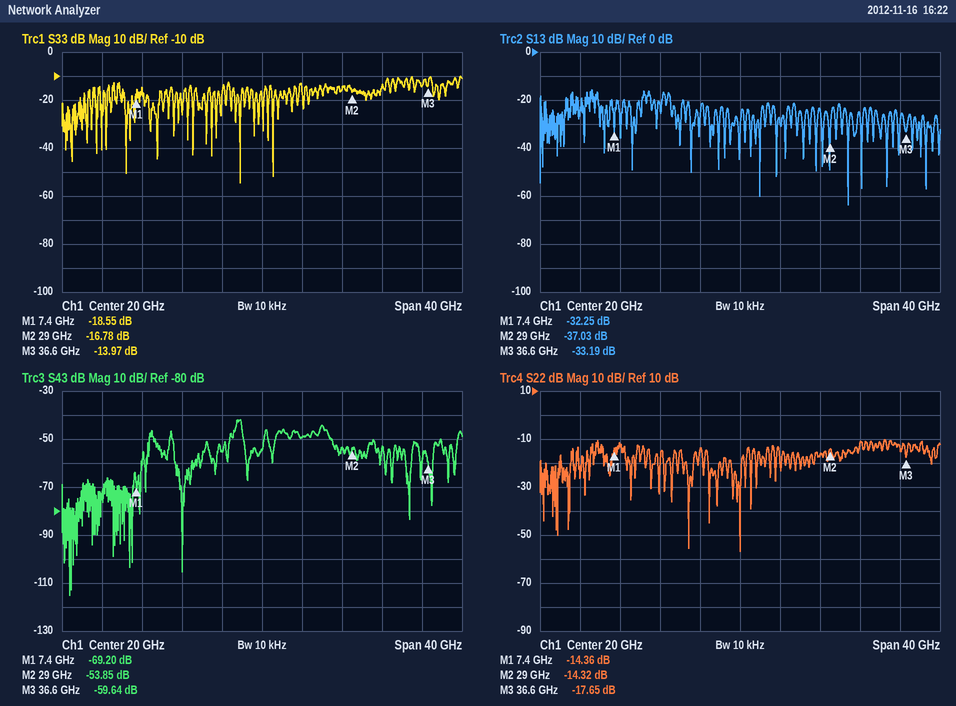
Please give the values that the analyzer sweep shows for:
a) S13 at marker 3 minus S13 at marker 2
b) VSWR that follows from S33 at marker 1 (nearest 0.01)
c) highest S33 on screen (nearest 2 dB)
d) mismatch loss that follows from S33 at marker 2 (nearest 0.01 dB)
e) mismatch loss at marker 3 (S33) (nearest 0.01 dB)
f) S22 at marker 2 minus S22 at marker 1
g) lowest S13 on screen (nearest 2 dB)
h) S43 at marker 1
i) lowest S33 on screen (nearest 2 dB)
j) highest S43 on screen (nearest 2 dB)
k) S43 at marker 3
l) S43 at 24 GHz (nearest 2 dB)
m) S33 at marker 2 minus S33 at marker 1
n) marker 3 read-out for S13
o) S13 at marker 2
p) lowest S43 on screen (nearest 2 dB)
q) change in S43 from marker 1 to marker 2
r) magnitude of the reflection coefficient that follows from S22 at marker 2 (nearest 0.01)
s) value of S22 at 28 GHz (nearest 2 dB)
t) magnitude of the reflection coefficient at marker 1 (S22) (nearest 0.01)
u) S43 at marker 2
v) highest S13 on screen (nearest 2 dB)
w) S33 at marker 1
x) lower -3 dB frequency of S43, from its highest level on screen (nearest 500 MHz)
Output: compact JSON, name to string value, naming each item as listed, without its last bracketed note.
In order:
{"S13 at marker 3 minus S13 at marker 2": "3.84 dB", "VSWR that follows from S33 at marker 1": "1.27", "highest S33 on screen": "-10 dB", "mismatch loss that follows from S33 at marker 2": "0.09 dB", "mismatch loss at marker 3 (S33)": "0.18 dB", "S22 at marker 2 minus S22 at marker 1": "0.04 dB", "lowest S13 on screen": "-64 dB", "S43 at marker 1": "-69.20 dB", "lowest S33 on screen": "-54 dB", "highest S43 on screen": "-42 dB", "S43 at marker 3": "-59.64 dB", "S43 at 24 GHz": "-50 dB", "S33 at marker 2 minus S33 at marker 1": "1.77 dB", "marker 3 read-out for S13": "-33.19 dB", "S13 at marker 2": "-37.03 dB", "lowest S43 on screen": "-116 dB", "change in S43 from marker 1 to marker 2": "15.35 dB", "magnitude of the reflection coefficient that follows from S22 at marker 2": "0.19", "value of S22 at 28 GHz": "-16 dB", "magnitude of the reflection coefficient at marker 1 (S22)": "0.19", "S43 at marker 2": "-53.85 dB", "highest S13 on screen": "-16 dB", "S33 at marker 1": "-18.55 dB", "lower -3 dB frequency of S43, from its highest level on screen": "17.5 GHz"}
